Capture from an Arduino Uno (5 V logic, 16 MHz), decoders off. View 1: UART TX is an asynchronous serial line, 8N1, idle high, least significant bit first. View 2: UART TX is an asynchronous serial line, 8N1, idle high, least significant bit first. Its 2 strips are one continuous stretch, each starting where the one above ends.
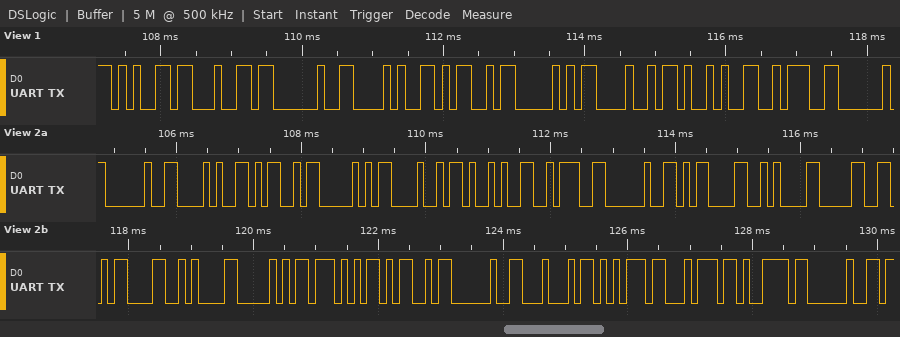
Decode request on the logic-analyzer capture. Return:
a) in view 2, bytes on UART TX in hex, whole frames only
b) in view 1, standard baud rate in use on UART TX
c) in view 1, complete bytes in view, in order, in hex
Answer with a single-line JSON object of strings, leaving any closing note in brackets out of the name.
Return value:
{"in view 2, bytes on UART TX in hex, whole frames only": "20 28 4D 50 48 29 3A 20 0D 0A 30 0D 0A 50 57 4D 20 44 75 74 79 20", "in view 1, standard baud rate in use on UART TX": "9600 baud", "in view 1, complete bytes in view, in order, in hex": "65 64 20 28 4D 50 48 29 3A"}
